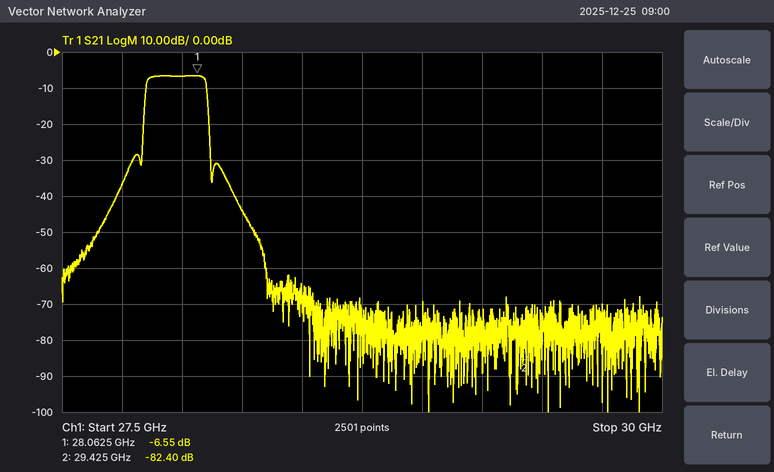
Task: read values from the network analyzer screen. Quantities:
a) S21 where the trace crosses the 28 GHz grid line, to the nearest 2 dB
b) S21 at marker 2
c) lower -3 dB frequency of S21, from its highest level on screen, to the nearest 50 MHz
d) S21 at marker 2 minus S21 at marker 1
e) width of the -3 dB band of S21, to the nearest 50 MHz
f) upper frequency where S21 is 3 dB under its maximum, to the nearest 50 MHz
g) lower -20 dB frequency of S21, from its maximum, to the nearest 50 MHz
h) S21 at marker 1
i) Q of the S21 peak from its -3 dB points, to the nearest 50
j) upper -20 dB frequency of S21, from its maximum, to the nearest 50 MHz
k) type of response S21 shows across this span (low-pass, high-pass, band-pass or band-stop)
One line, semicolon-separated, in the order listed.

-6 dB; -82.40 dB; 27.85 GHz; -75.85 dB; 250 MHz; 28.10 GHz; 27.85 GHz; -6.55 dB; 100; 28.10 GHz; band-pass
